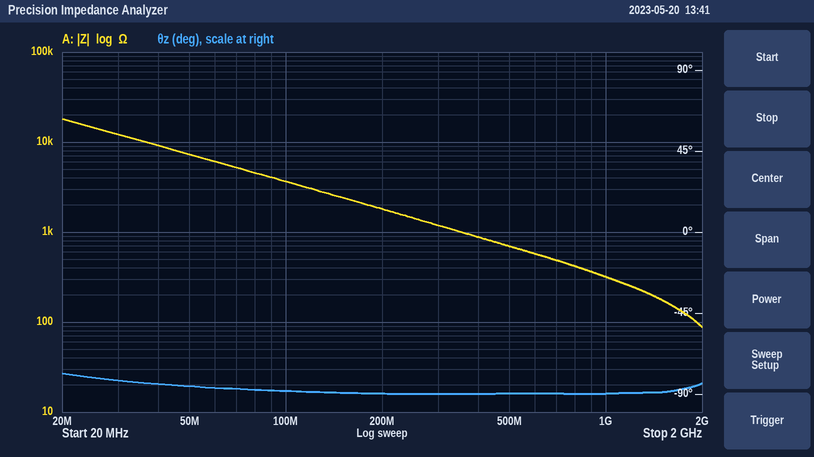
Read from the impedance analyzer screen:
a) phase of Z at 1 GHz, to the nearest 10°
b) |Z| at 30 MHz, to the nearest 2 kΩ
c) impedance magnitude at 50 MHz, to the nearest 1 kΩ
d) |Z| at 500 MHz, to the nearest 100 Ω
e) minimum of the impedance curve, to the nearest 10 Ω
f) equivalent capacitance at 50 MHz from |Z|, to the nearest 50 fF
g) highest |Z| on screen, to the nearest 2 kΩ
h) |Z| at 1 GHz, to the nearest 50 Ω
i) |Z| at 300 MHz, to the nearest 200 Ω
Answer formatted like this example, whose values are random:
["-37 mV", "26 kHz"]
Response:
["-90°", "12 kΩ", "7 kΩ", "700 Ω", "90 Ω", "450 fF", "18 kΩ", "300 Ω", "1.2 kΩ"]
